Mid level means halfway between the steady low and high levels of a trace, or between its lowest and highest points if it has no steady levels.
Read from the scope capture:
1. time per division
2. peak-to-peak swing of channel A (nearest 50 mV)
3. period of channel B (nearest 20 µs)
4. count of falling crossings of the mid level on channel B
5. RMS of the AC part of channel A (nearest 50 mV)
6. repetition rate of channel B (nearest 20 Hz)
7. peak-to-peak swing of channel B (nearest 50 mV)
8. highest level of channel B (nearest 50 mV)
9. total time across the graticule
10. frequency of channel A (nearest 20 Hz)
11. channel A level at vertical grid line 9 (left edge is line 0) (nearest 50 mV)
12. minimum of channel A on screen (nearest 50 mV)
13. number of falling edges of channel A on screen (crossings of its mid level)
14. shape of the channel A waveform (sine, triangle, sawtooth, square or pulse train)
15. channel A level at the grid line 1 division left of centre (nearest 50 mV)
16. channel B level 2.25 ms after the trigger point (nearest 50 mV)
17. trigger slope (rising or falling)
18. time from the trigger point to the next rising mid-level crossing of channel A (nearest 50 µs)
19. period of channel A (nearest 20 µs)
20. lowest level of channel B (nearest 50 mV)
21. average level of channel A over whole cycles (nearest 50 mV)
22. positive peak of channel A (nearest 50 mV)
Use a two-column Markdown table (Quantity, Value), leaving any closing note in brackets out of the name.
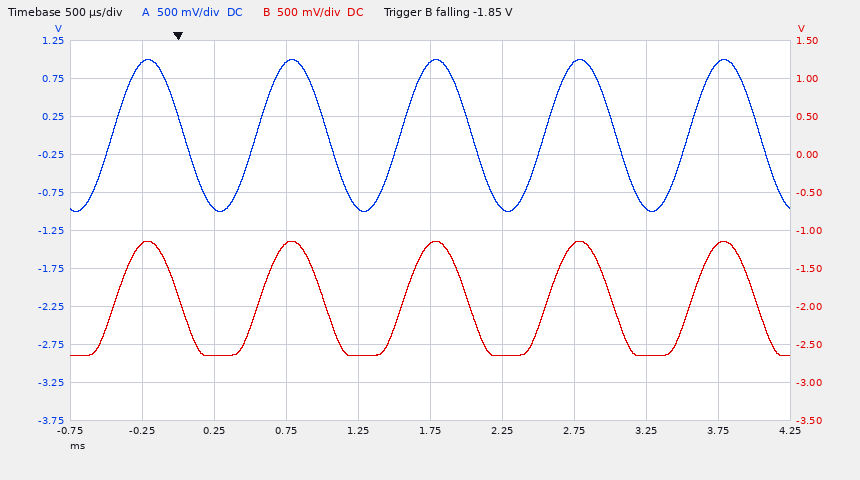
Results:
| Quantity | Value |
|---|---|
| time per division | 500 µs |
| peak-to-peak swing of channel A | 2.00 V |
| period of channel B | 1.00 ms |
| count of falling crossings of the mid level on channel B | 5 |
| RMS of the AC part of channel A | 700 mV |
| repetition rate of channel B | 1.00 kHz |
| peak-to-peak swing of channel B | 1.50 V |
| highest level of channel B | -1.15 V |
| total time across the graticule | 5 ms |
| frequency of channel A | 1.00 kHz |
| channel A level at vertical grid line 9 (left edge is line 0) | 950 mV |
| minimum of channel A on screen | -1.00 V |
| number of falling edges of channel A on screen | 5 |
| shape of the channel A waveform | sine |
| channel A level at the grid line 1 division left of centre | -950 mV |
| channel B level 2.25 ms after the trigger point | -2.65 V |
| trigger slope | falling |
| time from the trigger point to the next rising mid-level crossing of channel A | 550 µs |
| period of channel A | 1.00 ms |
| lowest level of channel B | -2.65 V |
| average level of channel A over whole cycles | 0 mV |
| positive peak of channel A | 1.00 V |
